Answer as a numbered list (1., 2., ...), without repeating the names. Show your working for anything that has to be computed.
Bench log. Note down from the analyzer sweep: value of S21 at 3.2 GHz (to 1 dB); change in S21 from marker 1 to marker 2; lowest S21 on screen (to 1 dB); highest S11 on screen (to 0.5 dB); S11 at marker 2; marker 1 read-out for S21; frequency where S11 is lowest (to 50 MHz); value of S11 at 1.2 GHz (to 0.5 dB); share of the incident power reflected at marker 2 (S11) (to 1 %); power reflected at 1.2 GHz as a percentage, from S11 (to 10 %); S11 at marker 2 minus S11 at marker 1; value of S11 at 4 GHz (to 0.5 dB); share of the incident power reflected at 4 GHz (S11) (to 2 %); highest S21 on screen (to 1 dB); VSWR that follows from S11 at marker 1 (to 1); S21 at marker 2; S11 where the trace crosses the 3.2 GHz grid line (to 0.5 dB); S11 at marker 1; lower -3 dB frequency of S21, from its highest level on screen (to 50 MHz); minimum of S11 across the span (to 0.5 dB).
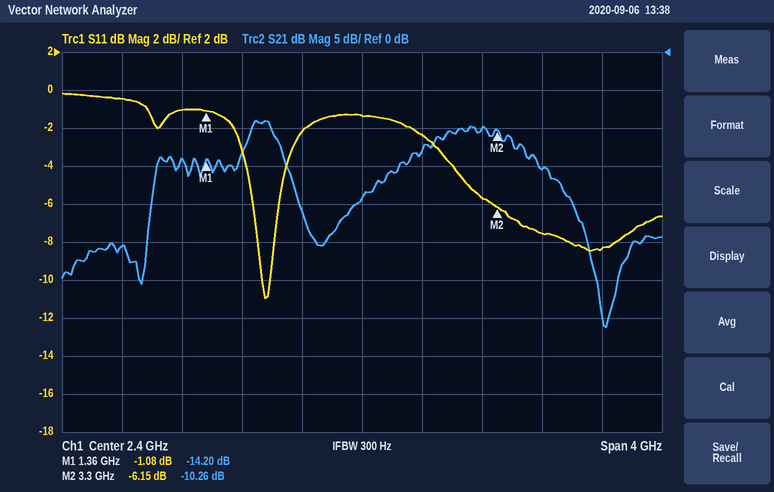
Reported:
1. -10 dB
2. -10.26 − (-14.2) = 3.94 dB
3. -36 dB
4. 0.0 dB
5. -6.15 dB
6. -14.20 dB
7. 1.75 GHz
8. -1.0 dB
9. 10^(-6.15/10) ≈ 24 %
10. 10^(-1/10) ≈ 79.4 %, so 80 % to the nearest 10 %
11. -6.15 − (-1.08) = -5.07 dB
12. -8.5 dB
13. 10^(-8.5/10) ≈ 14 %
14. -9 dB
15. (1 + 0.8831)/(1 − 0.8831) ≈ 16
16. -10.26 dB
17. -5.5 dB
18. -1.08 dB
19. 1.65 GHz
20. -11.0 dB
